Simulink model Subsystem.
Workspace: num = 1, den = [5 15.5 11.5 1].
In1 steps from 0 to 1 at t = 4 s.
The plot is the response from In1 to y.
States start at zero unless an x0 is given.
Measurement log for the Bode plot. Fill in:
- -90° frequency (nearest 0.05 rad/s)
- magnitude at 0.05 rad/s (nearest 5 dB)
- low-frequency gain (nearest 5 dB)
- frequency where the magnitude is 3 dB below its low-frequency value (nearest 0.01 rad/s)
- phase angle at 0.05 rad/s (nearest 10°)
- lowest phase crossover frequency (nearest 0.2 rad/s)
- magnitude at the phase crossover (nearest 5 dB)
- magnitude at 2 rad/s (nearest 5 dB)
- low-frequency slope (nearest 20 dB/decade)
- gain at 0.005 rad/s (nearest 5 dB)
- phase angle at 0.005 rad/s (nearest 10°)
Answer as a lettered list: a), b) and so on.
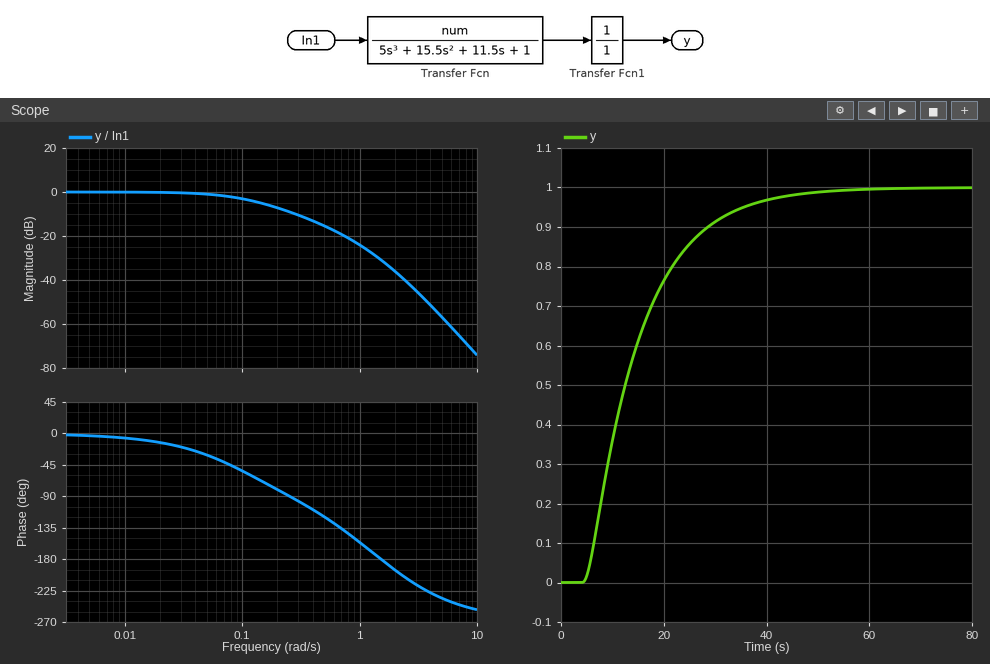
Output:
a) 0.25 rad/s
b) 0 dB
c) 0 dB
d) 0.10 rad/s
e) -30°
f) 1.6 rad/s
g) -30 dB
h) -35 dB
i) 0 dB/decade
j) 0 dB
k) 0°
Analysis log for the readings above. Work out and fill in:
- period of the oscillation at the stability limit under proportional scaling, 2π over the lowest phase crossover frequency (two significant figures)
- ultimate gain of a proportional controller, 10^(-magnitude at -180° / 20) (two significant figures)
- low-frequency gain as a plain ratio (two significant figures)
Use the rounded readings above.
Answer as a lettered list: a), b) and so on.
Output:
a) 3.9 s
b) 32
c) 1.0
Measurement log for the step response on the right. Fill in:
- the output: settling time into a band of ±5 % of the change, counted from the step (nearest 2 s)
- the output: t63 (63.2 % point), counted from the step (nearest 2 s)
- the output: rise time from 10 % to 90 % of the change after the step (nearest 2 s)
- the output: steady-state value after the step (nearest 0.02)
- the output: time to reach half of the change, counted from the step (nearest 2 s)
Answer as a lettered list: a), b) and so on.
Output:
a) 32 s
b) 12 s
c) 22 s
d) 1.00
e) 8 s
